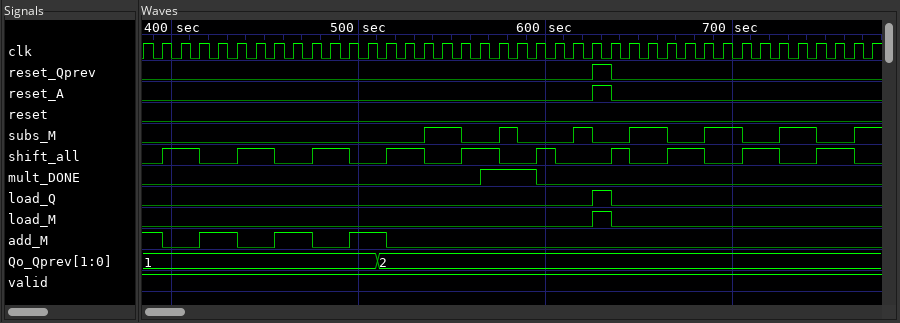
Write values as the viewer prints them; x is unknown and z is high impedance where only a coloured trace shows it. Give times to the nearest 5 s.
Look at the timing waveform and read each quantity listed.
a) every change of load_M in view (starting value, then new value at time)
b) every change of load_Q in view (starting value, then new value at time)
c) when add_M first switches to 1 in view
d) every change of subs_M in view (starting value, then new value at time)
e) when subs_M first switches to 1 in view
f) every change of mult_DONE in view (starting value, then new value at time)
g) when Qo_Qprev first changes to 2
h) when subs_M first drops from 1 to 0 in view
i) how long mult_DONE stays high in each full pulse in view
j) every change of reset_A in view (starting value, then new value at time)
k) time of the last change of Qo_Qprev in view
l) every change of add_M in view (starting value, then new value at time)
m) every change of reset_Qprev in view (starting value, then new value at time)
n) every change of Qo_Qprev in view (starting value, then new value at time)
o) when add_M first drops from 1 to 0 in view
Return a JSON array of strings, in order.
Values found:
["0, 1 at 625 s, 0 at 635 s", "0, 1 at 625 s, 0 at 635 s", "415 s", "0, 1 at 535 s, 0 at 555 s, 1 at 575 s, 0 at 585 s, 1 at 615 s, 0 at 625 s, 1 at 645 s, 0 at 665 s, 1 at 685 s, 0 at 705 s, 1 at 725 s, 0 at 745 s, 1 at 765 s", "535 s", "0, 1 at 565 s, 0 at 595 s", "510 s", "555 s", "30 s", "0, 1 at 625 s, 0 at 635 s", "510 s", "1, 0 at 395 s, 1 at 415 s, 0 at 435 s, 1 at 455 s, 0 at 475 s, 1 at 495 s, 0 at 515 s", "0, 1 at 625 s, 0 at 635 s", "1, 2 at 510 s", "395 s"]
